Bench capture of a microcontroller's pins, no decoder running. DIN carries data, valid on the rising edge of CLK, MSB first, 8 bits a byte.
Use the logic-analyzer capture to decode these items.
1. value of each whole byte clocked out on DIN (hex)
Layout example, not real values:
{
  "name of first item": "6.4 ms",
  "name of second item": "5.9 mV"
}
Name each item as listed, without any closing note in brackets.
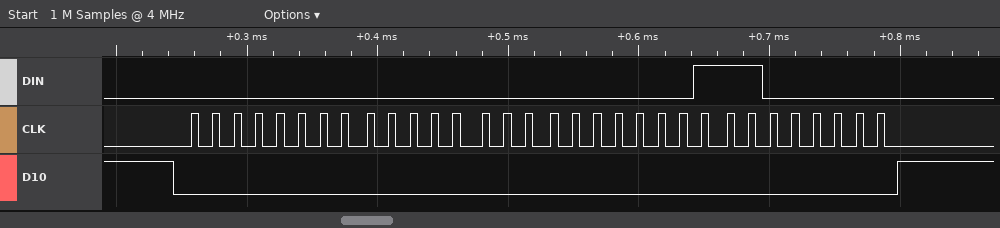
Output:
{
  "value of each whole byte clocked out on DIN": "00 00 01 C0"
}
